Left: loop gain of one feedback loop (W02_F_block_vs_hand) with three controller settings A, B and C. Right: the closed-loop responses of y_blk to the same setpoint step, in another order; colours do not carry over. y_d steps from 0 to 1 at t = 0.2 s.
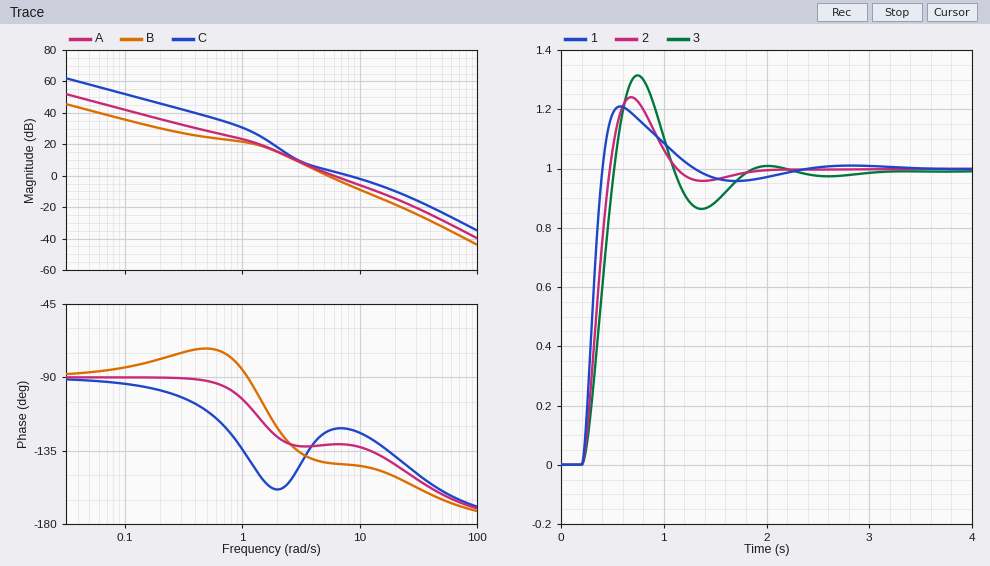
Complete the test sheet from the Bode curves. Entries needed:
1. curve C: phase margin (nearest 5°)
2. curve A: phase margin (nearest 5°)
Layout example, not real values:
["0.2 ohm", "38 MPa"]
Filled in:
["60°", "50°"]
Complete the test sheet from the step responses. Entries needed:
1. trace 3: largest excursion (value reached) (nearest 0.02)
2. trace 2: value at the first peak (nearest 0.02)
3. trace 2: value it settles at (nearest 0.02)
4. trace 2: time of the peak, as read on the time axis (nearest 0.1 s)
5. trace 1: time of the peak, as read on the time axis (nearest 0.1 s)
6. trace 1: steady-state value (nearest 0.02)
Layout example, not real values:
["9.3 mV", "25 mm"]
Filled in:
["1.32", "1.24", "1.00", "0.7 s", "0.6 s", "1.00"]
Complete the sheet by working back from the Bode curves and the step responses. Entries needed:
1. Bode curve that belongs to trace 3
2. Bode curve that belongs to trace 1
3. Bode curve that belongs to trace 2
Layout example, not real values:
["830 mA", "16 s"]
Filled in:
["B", "C", "A"]
